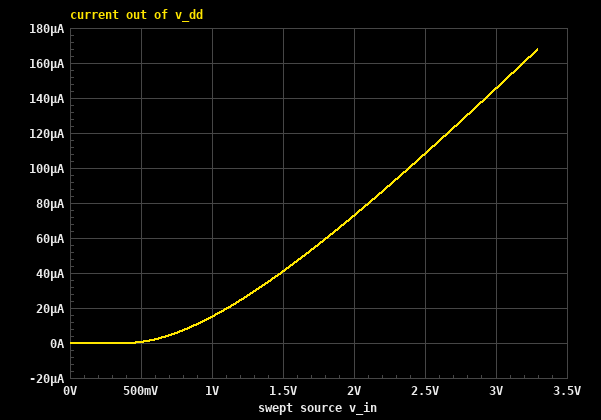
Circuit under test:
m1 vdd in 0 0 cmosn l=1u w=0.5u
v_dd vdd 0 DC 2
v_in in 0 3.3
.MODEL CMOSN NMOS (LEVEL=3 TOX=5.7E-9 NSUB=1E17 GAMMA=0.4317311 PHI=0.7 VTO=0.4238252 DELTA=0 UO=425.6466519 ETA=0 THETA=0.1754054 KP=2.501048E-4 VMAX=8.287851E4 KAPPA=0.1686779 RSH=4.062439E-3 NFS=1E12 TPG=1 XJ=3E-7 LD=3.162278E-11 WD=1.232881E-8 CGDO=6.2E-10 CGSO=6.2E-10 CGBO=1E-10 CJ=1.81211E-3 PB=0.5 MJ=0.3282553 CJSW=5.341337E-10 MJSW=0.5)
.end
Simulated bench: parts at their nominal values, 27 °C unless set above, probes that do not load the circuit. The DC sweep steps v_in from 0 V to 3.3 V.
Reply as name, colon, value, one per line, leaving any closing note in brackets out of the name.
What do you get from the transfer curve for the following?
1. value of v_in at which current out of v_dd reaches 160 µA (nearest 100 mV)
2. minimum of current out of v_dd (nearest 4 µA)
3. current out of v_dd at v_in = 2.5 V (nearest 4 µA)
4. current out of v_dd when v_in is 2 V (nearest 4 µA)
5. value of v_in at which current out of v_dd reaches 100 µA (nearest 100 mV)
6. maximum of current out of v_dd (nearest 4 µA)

value of v_in at which current out of v_dd reaches 160 µA: 3.2 V
minimum of current out of v_dd: 0 A
current out of v_dd at v_in = 2.5 V: 108 µA
current out of v_dd when v_in is 2 V: 72 µA
value of v_in at which current out of v_dd reaches 100 µA: 2.4 V
maximum of current out of v_dd: 168 µA
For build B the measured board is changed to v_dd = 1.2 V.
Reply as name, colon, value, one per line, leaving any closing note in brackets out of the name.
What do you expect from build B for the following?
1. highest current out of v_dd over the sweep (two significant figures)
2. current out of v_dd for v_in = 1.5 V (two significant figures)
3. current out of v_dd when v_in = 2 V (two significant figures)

highest current out of v_dd over the sweep: 150 µA
current out of v_dd for v_in = 1.5 V: 40 µA
current out of v_dd when v_in = 2 V: 71 µA
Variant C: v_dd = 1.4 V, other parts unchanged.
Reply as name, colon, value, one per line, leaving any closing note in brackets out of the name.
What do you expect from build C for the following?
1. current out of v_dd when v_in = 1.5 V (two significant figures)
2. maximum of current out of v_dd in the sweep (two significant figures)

current out of v_dd when v_in = 1.5 V: 40 µA
maximum of current out of v_dd in the sweep: 160 µA
